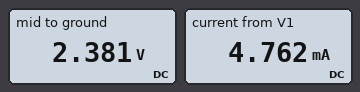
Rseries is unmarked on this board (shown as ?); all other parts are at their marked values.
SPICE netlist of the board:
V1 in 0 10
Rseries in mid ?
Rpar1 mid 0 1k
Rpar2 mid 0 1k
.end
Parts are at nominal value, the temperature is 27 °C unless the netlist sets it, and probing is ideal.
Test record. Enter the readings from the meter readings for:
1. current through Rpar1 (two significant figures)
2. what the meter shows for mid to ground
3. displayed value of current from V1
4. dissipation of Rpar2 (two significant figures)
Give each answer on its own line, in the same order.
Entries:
2.4 mA
2.381 V
4.762 mA
5.7 mW
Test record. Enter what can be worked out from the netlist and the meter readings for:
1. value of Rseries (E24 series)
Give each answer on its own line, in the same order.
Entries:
1.6 kΩ
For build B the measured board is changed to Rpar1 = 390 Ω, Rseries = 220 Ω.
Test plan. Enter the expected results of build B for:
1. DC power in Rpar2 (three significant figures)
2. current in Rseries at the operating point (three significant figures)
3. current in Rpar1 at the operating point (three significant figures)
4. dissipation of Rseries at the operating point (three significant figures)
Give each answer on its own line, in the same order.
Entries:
31.4 mW
20.0 mA
14.4 mA
87.8 mW
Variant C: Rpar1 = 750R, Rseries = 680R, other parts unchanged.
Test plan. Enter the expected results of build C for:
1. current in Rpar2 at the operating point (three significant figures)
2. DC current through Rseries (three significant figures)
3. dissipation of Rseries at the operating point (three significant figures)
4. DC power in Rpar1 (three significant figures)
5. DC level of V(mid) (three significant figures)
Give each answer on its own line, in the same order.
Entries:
3.87 mA
9.02 mA
55.3 mW
19.9 mW
3.87 V
